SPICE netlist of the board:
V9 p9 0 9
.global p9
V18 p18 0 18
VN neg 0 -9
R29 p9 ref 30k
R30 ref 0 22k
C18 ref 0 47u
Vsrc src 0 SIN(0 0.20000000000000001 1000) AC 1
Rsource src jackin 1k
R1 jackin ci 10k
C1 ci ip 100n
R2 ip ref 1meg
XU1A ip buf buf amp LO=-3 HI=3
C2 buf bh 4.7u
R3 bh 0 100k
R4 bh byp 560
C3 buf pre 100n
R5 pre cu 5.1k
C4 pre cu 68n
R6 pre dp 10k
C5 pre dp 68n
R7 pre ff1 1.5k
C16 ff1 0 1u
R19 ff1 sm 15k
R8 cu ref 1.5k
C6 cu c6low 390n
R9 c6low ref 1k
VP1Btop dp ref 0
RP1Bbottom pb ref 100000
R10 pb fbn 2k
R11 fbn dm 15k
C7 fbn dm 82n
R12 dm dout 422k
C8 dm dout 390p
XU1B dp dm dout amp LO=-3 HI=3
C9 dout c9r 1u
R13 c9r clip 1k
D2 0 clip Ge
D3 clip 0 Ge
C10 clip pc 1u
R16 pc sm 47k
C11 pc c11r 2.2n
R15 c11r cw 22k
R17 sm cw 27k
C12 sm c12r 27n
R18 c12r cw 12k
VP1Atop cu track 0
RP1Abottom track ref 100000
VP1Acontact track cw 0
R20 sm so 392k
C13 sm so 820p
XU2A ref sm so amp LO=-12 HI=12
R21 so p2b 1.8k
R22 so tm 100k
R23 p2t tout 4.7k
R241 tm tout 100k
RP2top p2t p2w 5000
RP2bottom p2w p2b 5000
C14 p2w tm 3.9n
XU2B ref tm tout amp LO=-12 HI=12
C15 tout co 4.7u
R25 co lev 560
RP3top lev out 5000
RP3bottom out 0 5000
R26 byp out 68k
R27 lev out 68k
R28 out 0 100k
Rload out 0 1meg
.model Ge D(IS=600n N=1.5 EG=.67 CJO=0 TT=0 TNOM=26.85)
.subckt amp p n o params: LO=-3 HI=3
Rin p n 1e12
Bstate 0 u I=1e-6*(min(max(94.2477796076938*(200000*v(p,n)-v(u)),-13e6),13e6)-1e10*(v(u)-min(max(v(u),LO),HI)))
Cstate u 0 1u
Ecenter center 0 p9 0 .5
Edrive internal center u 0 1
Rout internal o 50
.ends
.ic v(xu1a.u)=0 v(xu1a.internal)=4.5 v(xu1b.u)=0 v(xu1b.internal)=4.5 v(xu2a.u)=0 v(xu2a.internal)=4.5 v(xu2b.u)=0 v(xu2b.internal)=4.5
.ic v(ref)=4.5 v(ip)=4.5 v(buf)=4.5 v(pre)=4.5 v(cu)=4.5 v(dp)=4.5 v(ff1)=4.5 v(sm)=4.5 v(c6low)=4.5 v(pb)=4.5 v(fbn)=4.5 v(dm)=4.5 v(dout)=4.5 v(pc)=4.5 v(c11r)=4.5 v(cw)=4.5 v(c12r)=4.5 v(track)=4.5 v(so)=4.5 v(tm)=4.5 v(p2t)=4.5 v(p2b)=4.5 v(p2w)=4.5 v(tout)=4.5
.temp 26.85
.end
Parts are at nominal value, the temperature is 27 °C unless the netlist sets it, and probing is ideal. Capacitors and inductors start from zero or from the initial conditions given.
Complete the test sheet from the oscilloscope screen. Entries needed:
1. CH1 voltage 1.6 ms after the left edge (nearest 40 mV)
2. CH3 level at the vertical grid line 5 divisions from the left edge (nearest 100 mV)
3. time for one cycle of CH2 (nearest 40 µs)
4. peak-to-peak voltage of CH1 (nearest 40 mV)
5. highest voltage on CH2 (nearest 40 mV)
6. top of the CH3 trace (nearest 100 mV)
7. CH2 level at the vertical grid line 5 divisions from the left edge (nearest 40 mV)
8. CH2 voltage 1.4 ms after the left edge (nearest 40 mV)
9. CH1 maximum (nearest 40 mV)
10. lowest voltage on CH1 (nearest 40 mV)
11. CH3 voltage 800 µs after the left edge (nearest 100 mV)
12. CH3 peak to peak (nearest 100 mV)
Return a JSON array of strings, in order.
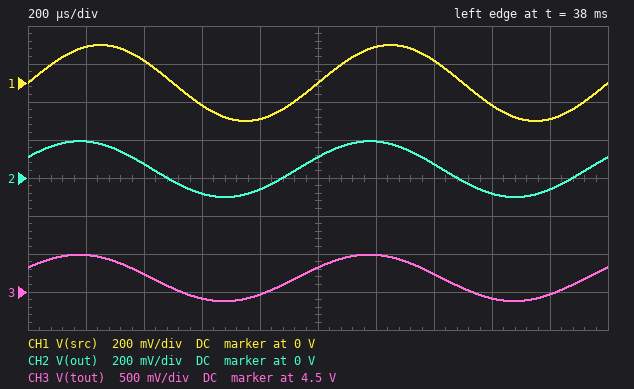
["-120 mV", "4.8 V", "1.00 ms", "400 mV", "200 mV", "5.0 V", "120 mV", "80 mV", "200 mV", "-200 mV", "4.5 V", "600 mV"]
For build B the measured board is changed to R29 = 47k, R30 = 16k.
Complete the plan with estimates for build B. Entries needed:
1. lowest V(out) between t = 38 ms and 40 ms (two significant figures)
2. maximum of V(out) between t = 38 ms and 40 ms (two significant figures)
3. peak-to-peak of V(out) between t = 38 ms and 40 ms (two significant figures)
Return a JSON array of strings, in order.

["47 mV", "340 mV", "290 mV"]
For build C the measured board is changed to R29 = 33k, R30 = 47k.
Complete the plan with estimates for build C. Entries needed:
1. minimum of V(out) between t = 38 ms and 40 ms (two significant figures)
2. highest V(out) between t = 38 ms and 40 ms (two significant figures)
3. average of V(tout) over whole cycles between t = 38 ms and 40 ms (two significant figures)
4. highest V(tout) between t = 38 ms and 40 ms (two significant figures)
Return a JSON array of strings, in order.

["-180 mV", "110 mV", "4.4 V", "4.7 V"]
